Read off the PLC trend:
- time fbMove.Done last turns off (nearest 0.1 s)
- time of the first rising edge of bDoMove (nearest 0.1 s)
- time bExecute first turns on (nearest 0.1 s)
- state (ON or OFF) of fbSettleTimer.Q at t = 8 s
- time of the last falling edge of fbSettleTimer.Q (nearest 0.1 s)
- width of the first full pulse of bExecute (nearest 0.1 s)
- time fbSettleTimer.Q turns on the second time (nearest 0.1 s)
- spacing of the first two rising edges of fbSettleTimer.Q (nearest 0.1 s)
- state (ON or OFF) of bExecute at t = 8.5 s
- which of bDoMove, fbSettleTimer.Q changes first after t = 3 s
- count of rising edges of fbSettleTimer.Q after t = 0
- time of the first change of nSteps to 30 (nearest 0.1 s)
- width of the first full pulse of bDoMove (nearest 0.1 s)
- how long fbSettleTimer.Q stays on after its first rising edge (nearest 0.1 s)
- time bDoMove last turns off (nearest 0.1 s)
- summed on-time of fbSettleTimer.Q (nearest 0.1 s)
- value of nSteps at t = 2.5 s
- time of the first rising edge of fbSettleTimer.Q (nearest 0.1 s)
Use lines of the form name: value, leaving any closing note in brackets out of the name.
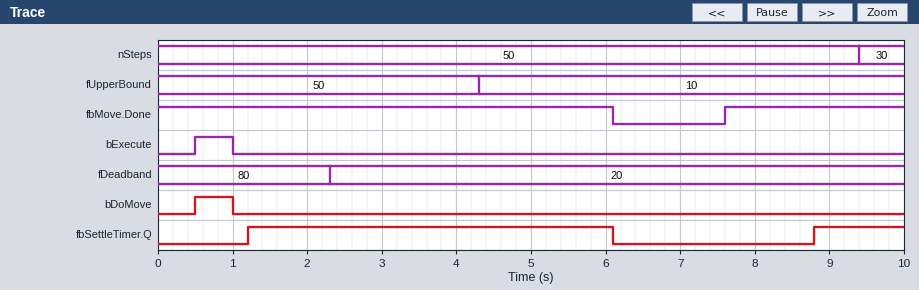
time fbMove.Done last turns off: 6.1 s
time of the first rising edge of bDoMove: 0.5 s
time bExecute first turns on: 0.5 s
state (ON or OFF) of fbSettleTimer.Q at t = 8 s: OFF
time of the last falling edge of fbSettleTimer.Q: 6.1 s
width of the first full pulse of bExecute: 0.5 s
time fbSettleTimer.Q turns on the second time: 8.8 s
spacing of the first two rising edges of fbSettleTimer.Q: 7.6 s
state (ON or OFF) of bExecute at t = 8.5 s: OFF
which of bDoMove, fbSettleTimer.Q changes first after t = 3 s: fbSettleTimer.Q
count of rising edges of fbSettleTimer.Q after t = 0: 2
time of the first change of nSteps to 30: 9.4 s
width of the first full pulse of bDoMove: 0.5 s
how long fbSettleTimer.Q stays on after its first rising edge: 4.9 s
time bDoMove last turns off: 1.0 s
summed on-time of fbSettleTimer.Q: 6.1 s
value of nSteps at t = 2.5 s: 50
time of the first rising edge of fbSettleTimer.Q: 1.2 s
